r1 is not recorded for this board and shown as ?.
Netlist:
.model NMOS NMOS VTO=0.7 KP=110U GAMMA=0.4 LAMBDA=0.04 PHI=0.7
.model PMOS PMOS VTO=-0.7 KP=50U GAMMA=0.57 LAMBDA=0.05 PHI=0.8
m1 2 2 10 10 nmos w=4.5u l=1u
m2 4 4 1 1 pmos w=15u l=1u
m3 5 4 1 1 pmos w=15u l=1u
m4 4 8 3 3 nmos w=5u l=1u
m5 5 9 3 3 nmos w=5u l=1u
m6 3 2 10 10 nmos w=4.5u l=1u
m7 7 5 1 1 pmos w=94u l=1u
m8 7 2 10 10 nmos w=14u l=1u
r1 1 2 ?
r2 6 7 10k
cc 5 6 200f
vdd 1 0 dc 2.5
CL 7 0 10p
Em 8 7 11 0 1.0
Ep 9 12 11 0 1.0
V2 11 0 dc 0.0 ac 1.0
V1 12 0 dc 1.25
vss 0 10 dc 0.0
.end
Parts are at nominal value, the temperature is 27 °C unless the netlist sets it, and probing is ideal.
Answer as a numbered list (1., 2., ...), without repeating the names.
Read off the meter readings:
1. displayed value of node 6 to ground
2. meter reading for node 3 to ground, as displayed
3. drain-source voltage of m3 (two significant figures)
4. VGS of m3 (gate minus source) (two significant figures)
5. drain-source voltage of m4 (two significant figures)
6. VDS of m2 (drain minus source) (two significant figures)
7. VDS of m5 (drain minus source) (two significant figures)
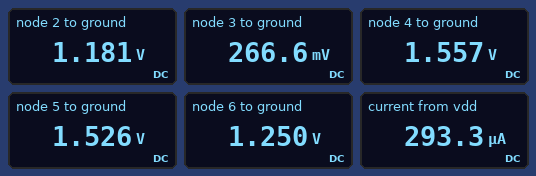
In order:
1. 1.250 V
2. 266.6 mV
3. -970 mV
4. -940 mV
5. 1.3 V
6. -940 mV
7. 1.3 V
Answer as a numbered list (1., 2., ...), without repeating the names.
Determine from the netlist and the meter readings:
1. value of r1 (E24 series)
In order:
1. 22 kΩ
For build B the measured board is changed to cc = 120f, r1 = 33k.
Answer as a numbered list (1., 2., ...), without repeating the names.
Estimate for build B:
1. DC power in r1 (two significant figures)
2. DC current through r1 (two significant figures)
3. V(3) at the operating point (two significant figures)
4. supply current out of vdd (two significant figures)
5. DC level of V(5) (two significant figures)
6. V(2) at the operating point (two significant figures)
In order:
1. 59 µW
2. 42 µA
3. 290 mV
4. 210 µA
5. 1.6 V
6. 1.1 V
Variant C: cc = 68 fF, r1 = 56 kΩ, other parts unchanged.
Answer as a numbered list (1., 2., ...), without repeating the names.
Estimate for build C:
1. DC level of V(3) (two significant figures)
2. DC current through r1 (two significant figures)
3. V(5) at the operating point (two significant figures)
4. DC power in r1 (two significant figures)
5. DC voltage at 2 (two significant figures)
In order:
1. 340 mV
2. 26 µA
3. 1.6 V
4. 39 µW
5. 1.0 V
